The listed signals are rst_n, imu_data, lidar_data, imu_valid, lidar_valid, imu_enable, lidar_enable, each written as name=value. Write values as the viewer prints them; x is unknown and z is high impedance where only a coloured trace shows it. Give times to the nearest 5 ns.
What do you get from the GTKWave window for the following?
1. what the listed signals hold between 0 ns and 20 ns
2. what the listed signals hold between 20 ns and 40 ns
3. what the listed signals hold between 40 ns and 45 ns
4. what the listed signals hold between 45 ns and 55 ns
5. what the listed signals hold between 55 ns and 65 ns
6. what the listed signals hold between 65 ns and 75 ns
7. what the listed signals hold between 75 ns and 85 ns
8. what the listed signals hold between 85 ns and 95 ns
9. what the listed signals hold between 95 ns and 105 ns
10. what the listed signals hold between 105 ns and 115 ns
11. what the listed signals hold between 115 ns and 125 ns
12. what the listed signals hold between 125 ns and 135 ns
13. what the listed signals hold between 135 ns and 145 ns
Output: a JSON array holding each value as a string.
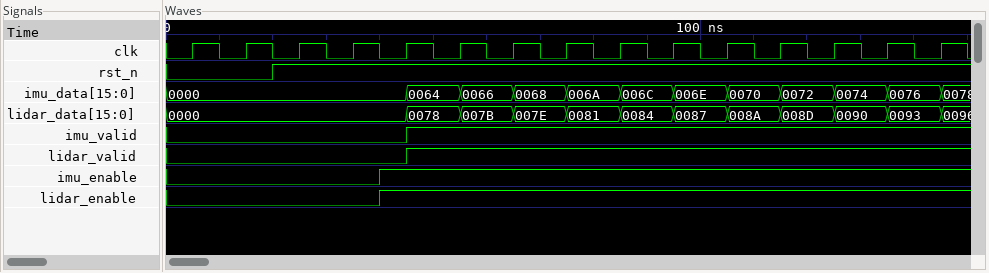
["rst_n=0, imu_data=0000, lidar_data=0000, imu_valid=0, lidar_valid=0, imu_enable=0, lidar_enable=0", "rst_n=1, imu_data=0000, lidar_data=0000, imu_valid=0, lidar_valid=0, imu_enable=0, lidar_enable=0", "rst_n=1, imu_data=0000, lidar_data=0000, imu_valid=0, lidar_valid=0, imu_enable=1, lidar_enable=1", "rst_n=1, imu_data=0064, lidar_data=0078, imu_valid=1, lidar_valid=1, imu_enable=1, lidar_enable=1", "rst_n=1, imu_data=0066, lidar_data=007B, imu_valid=1, lidar_valid=1, imu_enable=1, lidar_enable=1", "rst_n=1, imu_data=0068, lidar_data=007E, imu_valid=1, lidar_valid=1, imu_enable=1, lidar_enable=1", "rst_n=1, imu_data=006A, lidar_data=0081, imu_valid=1, lidar_valid=1, imu_enable=1, lidar_enable=1", "rst_n=1, imu_data=006C, lidar_data=0084, imu_valid=1, lidar_valid=1, imu_enable=1, lidar_enable=1", "rst_n=1, imu_data=006E, lidar_data=0087, imu_valid=1, lidar_valid=1, imu_enable=1, lidar_enable=1", "rst_n=1, imu_data=0070, lidar_data=008A, imu_valid=1, lidar_valid=1, imu_enable=1, lidar_enable=1", "rst_n=1, imu_data=0072, lidar_data=008D, imu_valid=1, lidar_valid=1, imu_enable=1, lidar_enable=1", "rst_n=1, imu_data=0074, lidar_data=0090, imu_valid=1, lidar_valid=1, imu_enable=1, lidar_enable=1", "rst_n=1, imu_data=0076, lidar_data=0093, imu_valid=1, lidar_valid=1, imu_enable=1, lidar_enable=1"]
